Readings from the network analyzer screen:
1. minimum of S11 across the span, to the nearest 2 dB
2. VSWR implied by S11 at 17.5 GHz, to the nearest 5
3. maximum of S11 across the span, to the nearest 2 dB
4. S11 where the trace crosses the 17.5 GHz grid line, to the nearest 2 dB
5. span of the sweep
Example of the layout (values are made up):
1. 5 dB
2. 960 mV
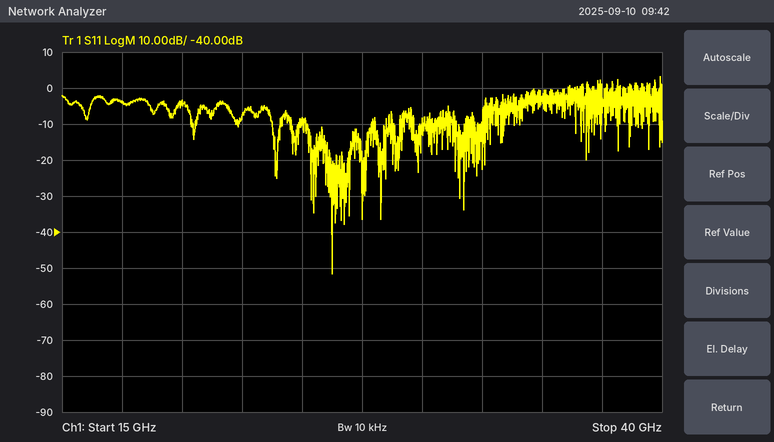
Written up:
1. -52 dB
2. 5
3. 4 dB
4. -4 dB
5. 25 GHz
